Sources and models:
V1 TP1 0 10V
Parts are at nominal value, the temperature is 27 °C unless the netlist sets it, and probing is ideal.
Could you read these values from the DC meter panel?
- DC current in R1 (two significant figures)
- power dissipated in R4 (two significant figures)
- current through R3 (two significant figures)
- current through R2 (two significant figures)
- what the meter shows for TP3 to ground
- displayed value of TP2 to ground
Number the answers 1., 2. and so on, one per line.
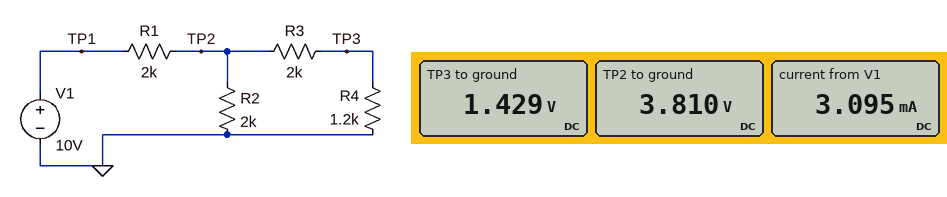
1. 3.1 mA
2. 1.7 mW
3. 1.2 mA
4. 1.9 mA
5. 1.429 V
6. 3.810 V
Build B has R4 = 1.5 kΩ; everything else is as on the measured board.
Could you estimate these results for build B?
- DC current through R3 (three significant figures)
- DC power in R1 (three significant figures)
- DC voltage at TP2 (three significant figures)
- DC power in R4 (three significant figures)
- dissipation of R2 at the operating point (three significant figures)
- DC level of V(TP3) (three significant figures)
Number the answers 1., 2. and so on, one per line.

1. 1.11 mA
2. 18.7 mW
3. 3.89 V
4. 1.85 mW
5. 7.56 mW
6. 1.67 V
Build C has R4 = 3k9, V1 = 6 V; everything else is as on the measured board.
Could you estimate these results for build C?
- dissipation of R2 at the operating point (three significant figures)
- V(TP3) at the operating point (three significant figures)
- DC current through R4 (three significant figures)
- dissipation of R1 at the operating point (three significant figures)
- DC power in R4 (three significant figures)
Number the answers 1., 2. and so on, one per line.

1. 3.29 mW
2. 1.70 V
3. 435 µA
4. 5.90 mW
5. 737 µW
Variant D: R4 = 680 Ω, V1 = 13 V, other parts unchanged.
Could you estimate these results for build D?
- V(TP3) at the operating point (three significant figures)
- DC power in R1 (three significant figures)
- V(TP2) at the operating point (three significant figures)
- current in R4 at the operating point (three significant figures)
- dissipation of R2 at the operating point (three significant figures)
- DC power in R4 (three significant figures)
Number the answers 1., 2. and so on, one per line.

1. 1.20 V
2. 34.2 mW
3. 4.73 V
4. 1.77 mA
5. 11.2 mW
6. 2.12 mW
